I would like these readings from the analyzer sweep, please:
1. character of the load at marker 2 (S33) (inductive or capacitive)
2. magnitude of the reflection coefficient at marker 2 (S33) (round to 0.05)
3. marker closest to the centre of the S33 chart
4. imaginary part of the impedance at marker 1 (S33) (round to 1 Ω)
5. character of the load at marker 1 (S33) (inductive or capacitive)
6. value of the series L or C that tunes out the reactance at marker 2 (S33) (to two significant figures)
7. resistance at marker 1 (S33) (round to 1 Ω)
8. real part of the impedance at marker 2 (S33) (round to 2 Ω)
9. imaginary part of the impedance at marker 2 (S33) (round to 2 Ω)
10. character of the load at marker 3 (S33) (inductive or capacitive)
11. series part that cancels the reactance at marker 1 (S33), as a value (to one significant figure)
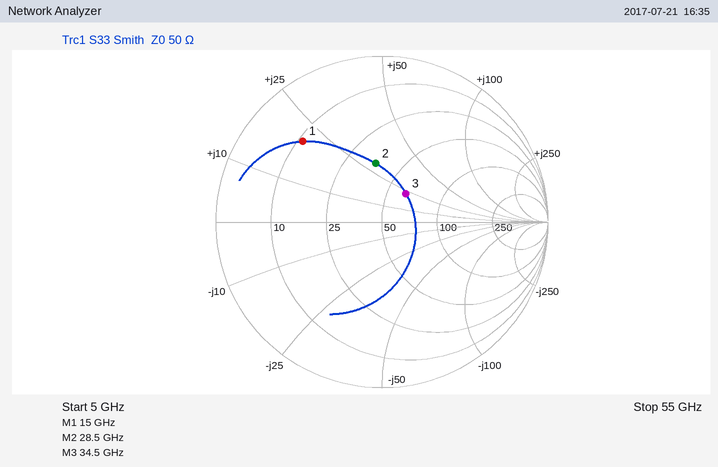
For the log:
inductive
0.35
marker 3
+20 Ω
inductive
190 fF
11 Ω
36 Ω
+30 Ω
inductive
500 fF
